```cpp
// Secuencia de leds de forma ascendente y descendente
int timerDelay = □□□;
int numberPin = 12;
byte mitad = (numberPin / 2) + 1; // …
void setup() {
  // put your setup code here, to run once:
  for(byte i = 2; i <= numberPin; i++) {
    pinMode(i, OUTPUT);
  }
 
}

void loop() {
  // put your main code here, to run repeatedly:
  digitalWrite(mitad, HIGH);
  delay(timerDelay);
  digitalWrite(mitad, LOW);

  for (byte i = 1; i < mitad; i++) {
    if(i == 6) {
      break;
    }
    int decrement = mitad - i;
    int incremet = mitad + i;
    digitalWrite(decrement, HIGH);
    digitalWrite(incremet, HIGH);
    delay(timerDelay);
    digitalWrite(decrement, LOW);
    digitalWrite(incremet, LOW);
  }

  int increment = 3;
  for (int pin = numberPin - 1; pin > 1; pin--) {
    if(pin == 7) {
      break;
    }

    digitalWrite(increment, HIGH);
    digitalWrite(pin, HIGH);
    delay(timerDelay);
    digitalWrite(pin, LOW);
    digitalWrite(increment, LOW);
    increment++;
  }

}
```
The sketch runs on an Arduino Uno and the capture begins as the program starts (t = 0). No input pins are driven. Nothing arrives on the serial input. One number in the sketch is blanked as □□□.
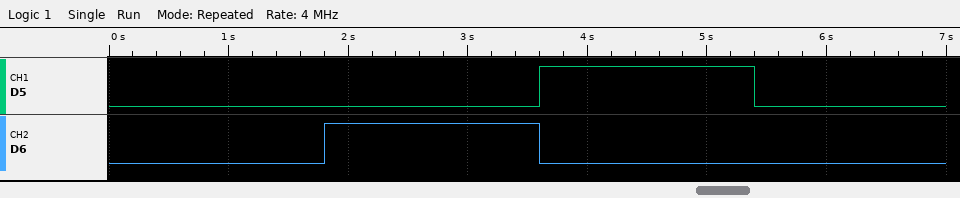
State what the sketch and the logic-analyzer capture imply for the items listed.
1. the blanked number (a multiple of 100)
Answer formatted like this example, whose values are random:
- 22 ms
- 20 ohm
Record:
- 1800
